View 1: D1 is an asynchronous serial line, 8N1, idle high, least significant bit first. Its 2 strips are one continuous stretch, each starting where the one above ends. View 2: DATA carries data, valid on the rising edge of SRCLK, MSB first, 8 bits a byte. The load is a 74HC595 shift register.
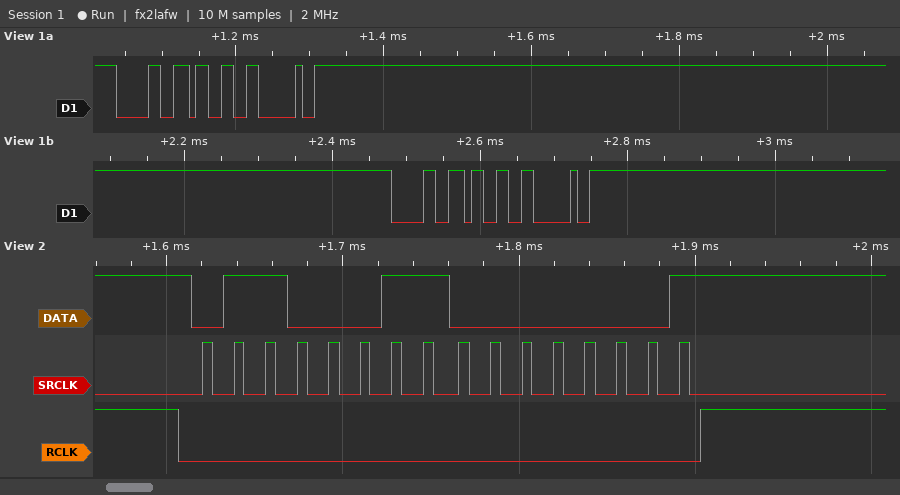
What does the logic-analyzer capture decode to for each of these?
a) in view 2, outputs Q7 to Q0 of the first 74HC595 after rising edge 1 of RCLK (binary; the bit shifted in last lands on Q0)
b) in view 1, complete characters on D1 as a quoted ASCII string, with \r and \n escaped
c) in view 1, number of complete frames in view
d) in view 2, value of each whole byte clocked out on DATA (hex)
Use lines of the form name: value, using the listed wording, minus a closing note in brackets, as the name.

in view 2, outputs Q7 to Q0 of the first 74HC595 after rising edge 1 of RCLK: 00000001
in view 1, complete characters on D1 as a quoted ASCII string, with \r and \n escaped: "03 03 "
in view 1, number of complete frames in view: 6
in view 2, value of each whole byte clocked out on DATA: 63 01
